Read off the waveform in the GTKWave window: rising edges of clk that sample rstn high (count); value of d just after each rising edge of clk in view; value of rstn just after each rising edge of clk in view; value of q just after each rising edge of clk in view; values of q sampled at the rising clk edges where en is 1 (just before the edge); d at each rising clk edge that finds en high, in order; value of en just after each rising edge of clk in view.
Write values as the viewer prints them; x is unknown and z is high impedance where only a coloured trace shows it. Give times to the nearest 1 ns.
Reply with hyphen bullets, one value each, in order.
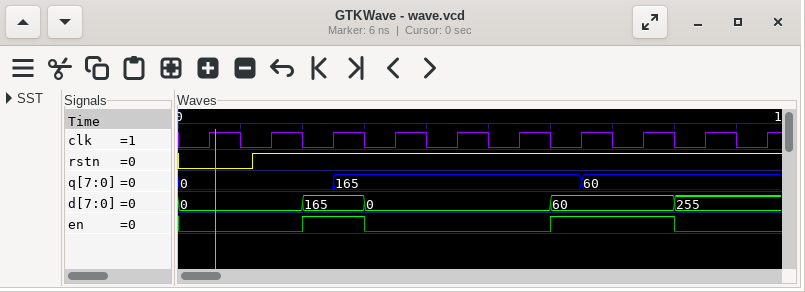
- 9
- 0, 0, 165, 0, 0, 0, 60, 60, 255, 255
- 0 1 1 1 1 1 1 1 1 1
- 0, 0, 165, 165, 165, 165, 60, 60, 60, 60
- 0, 165, 60
- 165, 60, 60
- 0 0 1 0 0 0 1 1 0 0
